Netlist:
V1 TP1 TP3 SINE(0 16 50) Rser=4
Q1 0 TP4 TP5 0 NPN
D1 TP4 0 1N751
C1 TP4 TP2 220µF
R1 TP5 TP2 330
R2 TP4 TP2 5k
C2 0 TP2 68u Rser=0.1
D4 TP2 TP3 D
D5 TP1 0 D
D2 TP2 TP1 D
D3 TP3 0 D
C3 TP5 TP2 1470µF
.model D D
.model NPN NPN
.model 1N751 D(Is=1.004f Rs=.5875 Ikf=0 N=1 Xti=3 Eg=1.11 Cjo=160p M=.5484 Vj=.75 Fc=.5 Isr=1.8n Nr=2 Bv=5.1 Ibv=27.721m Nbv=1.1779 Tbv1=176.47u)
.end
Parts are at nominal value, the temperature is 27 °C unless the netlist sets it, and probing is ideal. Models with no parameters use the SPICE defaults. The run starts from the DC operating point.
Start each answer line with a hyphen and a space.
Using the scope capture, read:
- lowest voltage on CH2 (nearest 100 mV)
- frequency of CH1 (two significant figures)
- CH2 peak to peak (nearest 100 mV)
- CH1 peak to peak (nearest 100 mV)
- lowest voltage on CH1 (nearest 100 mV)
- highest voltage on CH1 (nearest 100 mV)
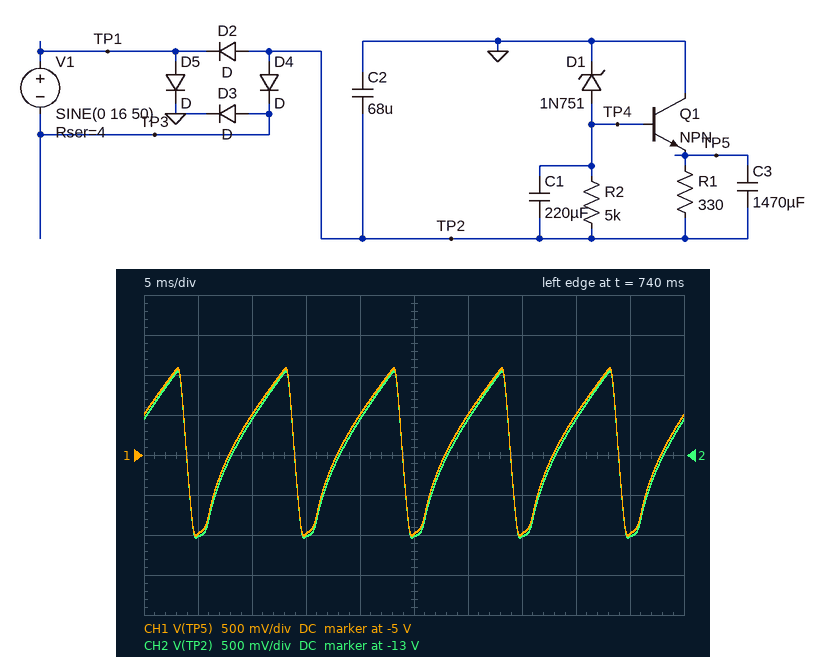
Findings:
- -14.0 V
- 100 Hz
- 2.1 V
- 2.1 V
- -6.0 V
- -3.9 V
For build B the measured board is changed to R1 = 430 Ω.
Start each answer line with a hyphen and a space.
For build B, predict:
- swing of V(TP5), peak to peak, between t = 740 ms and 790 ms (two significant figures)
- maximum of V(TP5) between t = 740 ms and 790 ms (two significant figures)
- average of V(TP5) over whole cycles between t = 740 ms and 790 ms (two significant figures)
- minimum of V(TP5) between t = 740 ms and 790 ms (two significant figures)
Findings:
- 1.7 V
- -4.3 V
- -5.0 V
- -6.0 V
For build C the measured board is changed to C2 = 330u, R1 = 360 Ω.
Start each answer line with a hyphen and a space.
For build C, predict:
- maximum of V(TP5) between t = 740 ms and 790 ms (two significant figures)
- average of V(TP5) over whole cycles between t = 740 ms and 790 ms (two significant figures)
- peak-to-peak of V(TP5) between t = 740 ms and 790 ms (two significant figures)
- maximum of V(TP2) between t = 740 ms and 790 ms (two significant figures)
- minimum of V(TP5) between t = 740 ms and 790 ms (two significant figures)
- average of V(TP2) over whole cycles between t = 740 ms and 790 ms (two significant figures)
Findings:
- -5.5 V
- -5.7 V
- 500 mV
- -13 V
- -6.0 V
- -14 V
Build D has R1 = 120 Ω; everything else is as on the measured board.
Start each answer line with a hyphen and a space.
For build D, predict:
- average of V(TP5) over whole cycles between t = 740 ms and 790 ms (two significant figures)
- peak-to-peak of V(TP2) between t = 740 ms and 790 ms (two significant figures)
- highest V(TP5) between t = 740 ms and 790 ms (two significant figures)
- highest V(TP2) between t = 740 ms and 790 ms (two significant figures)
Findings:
- -3.9 V
- 4.8 V
- -1.2 V
- -8.9 V
